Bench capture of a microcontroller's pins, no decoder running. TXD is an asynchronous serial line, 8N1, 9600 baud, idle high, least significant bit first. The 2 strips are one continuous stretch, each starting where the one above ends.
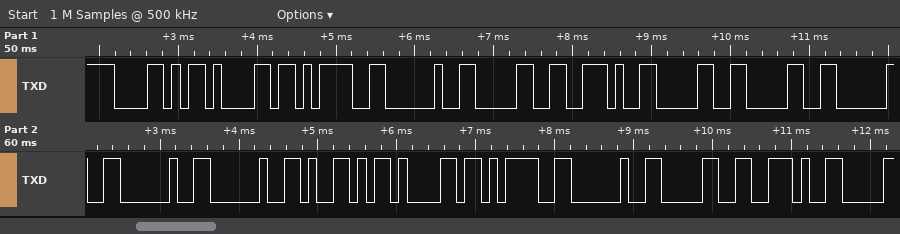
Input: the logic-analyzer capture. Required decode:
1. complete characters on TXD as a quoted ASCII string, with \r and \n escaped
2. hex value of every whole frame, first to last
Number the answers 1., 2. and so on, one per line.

1. "Xa= 0.00   Ya= 0."
2. 0x58 0x61 0x3D 0x20 0x30 0x2E 0x30 0x30 0x20 0x20 0x20 0x59 0x61 0x3D 0x20 0x30 0x2E
